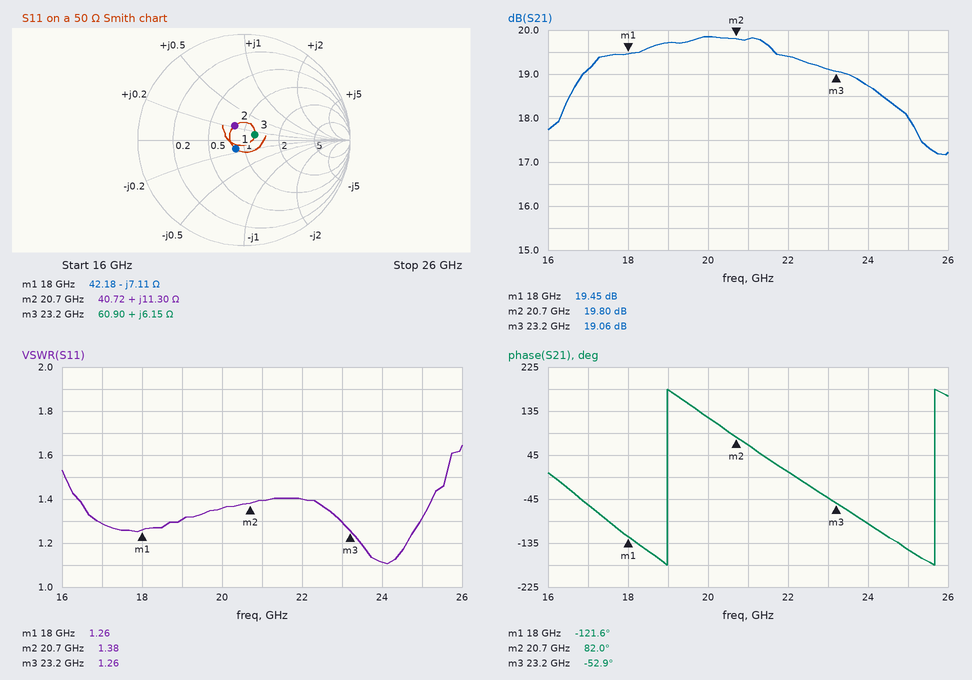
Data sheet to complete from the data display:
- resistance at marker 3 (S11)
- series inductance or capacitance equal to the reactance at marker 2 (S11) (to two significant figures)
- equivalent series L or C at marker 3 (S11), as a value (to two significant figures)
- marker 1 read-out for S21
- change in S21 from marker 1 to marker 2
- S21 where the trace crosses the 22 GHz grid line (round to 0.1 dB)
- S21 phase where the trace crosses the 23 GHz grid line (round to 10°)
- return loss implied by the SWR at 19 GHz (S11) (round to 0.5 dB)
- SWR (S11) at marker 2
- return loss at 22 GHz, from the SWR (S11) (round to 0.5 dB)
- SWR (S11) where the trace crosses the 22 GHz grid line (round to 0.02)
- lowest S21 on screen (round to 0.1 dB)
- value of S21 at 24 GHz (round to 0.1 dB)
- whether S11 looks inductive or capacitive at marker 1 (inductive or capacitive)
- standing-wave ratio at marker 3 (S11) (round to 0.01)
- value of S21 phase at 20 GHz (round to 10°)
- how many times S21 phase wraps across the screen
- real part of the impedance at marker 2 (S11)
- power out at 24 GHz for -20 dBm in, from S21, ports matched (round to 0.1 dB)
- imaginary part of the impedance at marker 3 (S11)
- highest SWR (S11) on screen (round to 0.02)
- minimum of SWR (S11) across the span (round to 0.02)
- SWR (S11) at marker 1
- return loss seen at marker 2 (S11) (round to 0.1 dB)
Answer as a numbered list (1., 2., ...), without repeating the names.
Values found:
1. 60.90 Ω
2. 87 pH
3. 42 pH
4. 19.45 dB
5. 0.35 dB
6. 19.4 dB
7. -40°
8. 17.5 dB
9. 1.38
10. 15.5 dB
11. 1.40
12. 17.2 dB
13. 18.7 dB
14. capacitive
15. 1.25
16. 120°
17. 2
18. 40.72 Ω
19. -1.3 dBm
20. +6.15 Ω
21. 1.64
22. 1.10
23. 1.26
24. 15.9 dB
